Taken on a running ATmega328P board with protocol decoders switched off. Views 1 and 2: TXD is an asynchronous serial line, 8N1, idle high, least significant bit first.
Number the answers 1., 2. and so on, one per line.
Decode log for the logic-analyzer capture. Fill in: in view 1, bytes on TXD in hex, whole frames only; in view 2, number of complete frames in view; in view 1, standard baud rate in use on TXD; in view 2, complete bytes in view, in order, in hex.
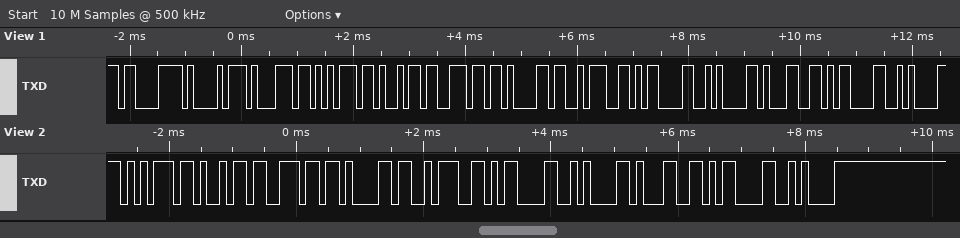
1. C3 A1 71 75 69 6E 61 3A 0D 0A 31 0D 0A
2. 10
3. 9600 baud
4. 75 69 6E 61 3A 0D 0A 31 0D 0A
